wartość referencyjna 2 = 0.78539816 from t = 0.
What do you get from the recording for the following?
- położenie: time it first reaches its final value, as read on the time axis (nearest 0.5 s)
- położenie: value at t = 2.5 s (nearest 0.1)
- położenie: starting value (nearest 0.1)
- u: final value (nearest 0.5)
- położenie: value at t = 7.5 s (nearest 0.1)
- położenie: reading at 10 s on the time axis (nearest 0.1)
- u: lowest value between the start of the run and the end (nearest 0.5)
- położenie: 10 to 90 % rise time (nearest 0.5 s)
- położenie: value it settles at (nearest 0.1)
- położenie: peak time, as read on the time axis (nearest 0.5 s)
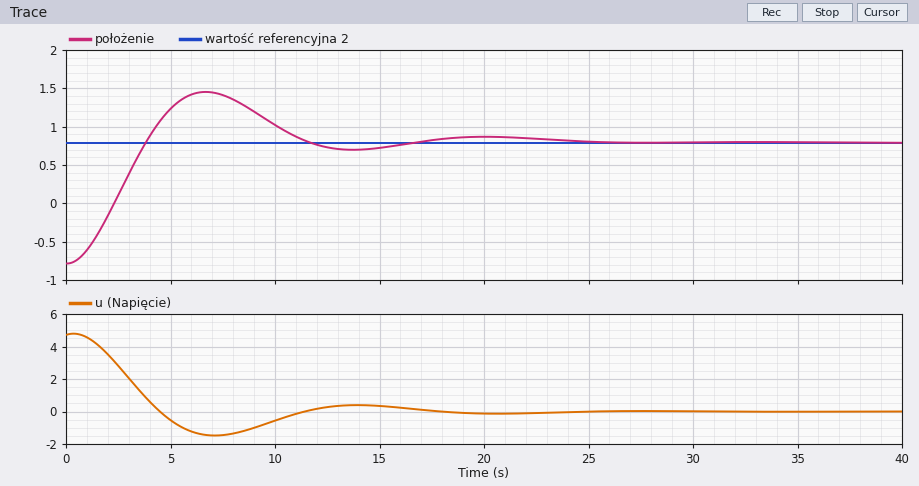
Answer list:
4.0 s
0.1
-0.8
0.0
1.4
1.0
-1.5
2.5 s
0.8
6.5 s
